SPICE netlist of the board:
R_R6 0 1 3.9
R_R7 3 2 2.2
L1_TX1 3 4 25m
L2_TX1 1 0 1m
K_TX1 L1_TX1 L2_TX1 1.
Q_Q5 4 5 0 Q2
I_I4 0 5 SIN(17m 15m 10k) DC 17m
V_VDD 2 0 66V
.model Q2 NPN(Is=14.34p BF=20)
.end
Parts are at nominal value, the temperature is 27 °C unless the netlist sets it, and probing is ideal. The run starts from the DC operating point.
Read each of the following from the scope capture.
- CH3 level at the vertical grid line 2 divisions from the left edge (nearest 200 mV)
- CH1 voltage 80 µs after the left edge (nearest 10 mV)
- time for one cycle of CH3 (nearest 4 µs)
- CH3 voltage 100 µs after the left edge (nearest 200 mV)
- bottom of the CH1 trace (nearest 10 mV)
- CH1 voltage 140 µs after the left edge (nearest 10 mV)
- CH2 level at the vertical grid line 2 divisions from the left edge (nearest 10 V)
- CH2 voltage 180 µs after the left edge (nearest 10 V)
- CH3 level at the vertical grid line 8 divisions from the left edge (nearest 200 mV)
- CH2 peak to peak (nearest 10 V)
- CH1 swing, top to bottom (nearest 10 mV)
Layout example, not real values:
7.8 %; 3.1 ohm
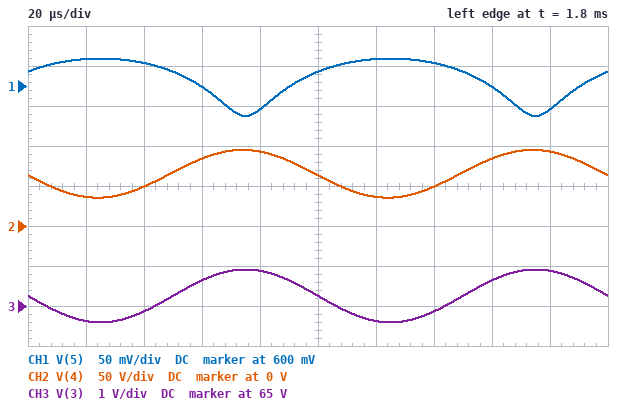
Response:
64.8 V; 570 mV; 100 µs; 65.2 V; 560 mV; 630 mV; 50 V; 90 V; 65.6 V; 60 V; 70 mV
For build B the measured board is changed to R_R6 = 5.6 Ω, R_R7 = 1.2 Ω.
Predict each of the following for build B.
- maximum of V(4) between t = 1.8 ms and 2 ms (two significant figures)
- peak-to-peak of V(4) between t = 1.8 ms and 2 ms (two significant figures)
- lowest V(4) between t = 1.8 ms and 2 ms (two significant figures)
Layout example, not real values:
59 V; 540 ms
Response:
110 V; 84 V; 23 V
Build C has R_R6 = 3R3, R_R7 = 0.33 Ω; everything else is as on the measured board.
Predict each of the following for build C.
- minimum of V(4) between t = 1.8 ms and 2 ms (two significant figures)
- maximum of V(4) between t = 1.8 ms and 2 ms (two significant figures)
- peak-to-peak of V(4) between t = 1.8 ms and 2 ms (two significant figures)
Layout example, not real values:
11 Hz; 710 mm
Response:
41 V; 91 V; 50 V
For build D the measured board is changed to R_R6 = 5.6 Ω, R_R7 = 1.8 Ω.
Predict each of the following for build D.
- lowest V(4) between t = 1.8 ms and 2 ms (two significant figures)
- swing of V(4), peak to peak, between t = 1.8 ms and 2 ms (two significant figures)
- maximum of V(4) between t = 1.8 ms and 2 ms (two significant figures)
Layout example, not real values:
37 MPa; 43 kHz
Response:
23 V; 85 V; 110 V
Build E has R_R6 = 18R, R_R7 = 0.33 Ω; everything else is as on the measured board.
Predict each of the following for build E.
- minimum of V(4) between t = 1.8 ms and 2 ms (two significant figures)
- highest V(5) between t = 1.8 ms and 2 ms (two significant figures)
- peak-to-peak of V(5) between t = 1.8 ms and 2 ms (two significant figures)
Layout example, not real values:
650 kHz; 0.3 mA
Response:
100 mV; 630 mV; 65 mV
